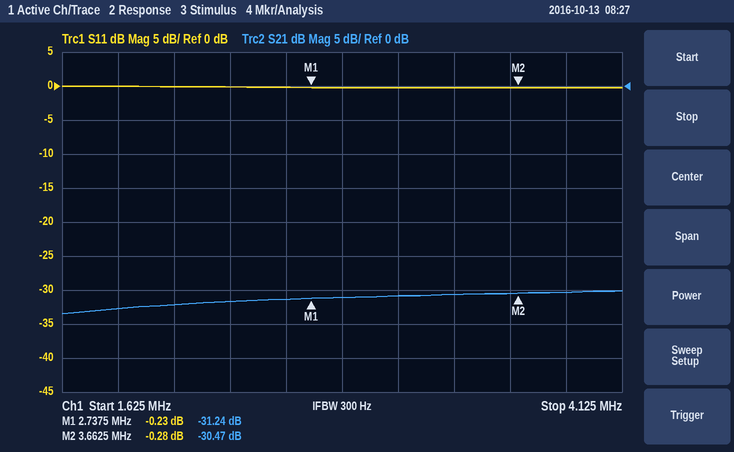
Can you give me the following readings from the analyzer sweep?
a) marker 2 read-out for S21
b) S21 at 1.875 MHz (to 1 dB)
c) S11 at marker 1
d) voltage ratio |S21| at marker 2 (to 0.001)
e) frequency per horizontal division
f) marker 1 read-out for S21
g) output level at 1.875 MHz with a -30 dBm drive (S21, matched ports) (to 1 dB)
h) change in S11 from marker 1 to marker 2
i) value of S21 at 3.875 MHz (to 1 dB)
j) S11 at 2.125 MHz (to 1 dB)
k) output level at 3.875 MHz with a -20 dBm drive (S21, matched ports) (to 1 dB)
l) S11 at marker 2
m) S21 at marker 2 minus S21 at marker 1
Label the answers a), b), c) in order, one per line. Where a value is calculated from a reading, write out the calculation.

a) -30.47 dB
b) -33 dB
c) -0.23 dB
d) 10^(-30.47/20) ≈ 0.030
e) 250 kHz
f) -31.24 dB
g) -30 dBm + (-33 dB) = -63 dBm
h) -0.28 − (-0.23) = -0.05 dB
i) -30 dB
j) 0 dB
k) -20 dBm + (-30 dB) = -50 dBm
l) -0.28 dB
m) -30.47 − (-31.24) = 0.77 dB
